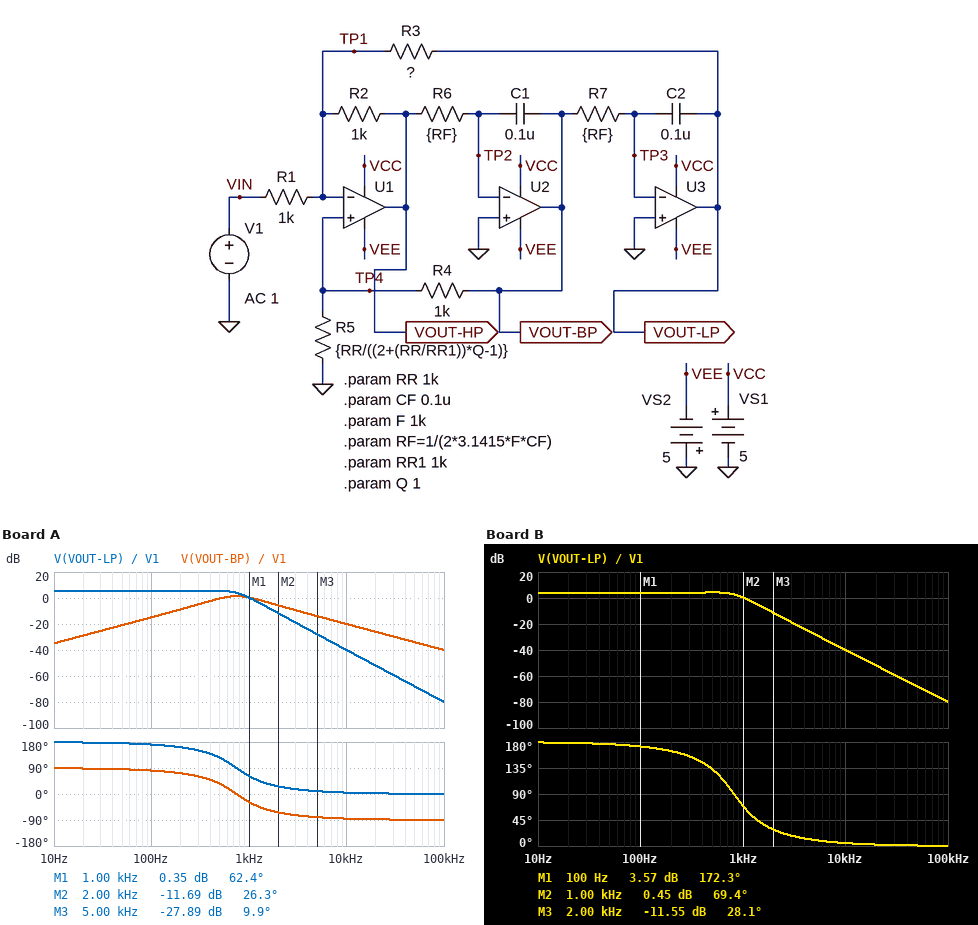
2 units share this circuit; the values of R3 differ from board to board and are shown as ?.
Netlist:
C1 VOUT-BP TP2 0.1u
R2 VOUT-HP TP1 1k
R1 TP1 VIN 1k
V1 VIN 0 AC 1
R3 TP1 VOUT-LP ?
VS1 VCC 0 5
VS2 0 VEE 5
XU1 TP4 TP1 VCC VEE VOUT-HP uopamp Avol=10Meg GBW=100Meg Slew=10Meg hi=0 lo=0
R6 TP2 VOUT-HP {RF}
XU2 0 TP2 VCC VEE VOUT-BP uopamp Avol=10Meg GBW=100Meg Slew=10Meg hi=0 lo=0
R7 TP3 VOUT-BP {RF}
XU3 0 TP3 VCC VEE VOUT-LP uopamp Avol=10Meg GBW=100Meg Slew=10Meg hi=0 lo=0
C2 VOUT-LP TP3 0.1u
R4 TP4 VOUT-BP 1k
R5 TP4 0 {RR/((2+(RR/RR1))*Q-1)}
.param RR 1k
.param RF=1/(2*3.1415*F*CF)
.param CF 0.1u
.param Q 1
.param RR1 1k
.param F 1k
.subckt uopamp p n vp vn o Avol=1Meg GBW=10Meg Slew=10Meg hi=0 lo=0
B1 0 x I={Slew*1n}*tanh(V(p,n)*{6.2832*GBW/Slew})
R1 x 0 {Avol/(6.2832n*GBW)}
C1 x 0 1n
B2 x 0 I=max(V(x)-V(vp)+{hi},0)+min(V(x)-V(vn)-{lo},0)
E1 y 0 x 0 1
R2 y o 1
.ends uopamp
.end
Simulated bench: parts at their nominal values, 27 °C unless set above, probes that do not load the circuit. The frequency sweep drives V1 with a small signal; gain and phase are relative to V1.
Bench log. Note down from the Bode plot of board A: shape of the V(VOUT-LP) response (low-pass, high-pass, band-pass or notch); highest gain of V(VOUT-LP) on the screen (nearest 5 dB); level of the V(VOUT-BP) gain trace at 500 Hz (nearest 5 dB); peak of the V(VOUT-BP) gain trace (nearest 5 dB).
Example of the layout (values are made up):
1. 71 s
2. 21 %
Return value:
1. low-pass
2. 5 dB
3. 0 dB
4. 0 dB
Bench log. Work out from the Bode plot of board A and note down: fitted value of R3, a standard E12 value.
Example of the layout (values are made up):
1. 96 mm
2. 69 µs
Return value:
1. 1.8 kΩ
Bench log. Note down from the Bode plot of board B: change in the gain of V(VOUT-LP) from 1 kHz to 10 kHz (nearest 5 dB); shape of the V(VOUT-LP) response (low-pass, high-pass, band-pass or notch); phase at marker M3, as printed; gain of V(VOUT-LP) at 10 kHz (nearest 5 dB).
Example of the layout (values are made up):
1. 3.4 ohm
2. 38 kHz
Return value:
1. -40 dB
2. low-pass
3. 28.1 deg
4. -40 dB
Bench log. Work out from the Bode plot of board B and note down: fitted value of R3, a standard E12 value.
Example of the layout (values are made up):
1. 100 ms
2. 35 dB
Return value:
1. 1.5 kΩ
